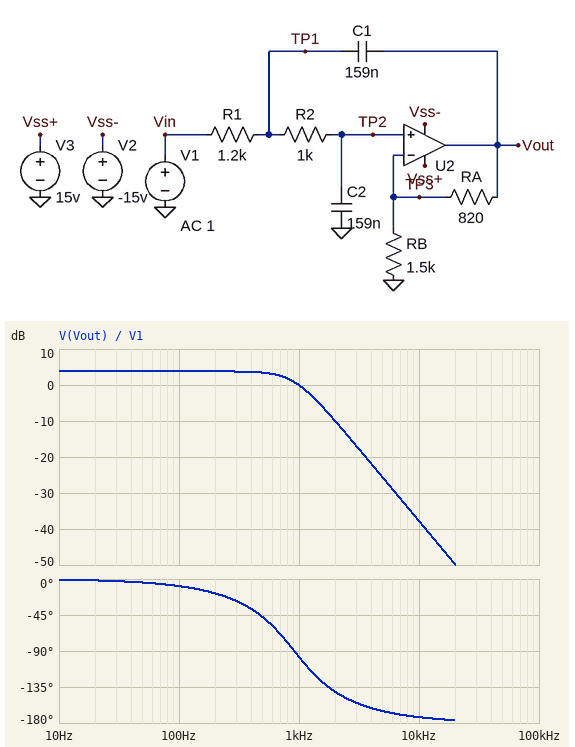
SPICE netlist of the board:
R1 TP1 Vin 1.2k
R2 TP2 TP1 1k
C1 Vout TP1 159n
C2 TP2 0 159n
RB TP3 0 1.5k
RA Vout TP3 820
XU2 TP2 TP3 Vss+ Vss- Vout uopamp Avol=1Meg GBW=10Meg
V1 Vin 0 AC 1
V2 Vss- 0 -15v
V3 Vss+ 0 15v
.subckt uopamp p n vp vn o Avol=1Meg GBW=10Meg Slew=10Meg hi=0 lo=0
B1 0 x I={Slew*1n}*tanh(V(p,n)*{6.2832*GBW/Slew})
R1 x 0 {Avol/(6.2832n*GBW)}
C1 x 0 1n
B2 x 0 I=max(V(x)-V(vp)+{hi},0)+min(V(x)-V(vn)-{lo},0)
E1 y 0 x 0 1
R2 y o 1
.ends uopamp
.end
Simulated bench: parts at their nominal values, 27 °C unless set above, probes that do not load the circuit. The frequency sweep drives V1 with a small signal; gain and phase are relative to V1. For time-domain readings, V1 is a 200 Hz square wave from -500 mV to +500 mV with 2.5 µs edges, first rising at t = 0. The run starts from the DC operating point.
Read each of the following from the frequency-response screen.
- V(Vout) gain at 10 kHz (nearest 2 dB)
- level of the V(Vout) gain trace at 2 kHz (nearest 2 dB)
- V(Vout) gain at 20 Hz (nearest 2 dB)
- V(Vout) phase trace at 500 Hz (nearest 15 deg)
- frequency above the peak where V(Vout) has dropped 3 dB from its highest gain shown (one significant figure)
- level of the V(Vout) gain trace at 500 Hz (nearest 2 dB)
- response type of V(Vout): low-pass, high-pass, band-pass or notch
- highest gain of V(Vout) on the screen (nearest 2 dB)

-38 dB
-10 dB
4 dB
-45 deg
900 Hz
4 dB
low-pass
4 dB
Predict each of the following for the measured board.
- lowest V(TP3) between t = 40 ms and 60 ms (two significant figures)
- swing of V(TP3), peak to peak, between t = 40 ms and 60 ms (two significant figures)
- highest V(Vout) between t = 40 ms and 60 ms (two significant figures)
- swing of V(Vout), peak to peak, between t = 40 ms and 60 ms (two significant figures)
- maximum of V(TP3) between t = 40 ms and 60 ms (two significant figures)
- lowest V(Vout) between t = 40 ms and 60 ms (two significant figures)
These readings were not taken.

-540 mV
1.1 V
840 mV
1.7 V
540 mV
-840 mV
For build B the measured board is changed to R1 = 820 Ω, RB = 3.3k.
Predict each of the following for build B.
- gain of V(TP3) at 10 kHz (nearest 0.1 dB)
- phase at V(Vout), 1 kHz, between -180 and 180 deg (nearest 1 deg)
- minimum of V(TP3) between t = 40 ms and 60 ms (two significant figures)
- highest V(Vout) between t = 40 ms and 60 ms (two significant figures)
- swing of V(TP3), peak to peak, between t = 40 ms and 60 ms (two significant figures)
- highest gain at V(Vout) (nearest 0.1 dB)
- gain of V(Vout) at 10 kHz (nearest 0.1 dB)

-38.3 dB
-84 deg
-500 mV
630 mV
1.0 V
1.9 dB
-36.4 dB
